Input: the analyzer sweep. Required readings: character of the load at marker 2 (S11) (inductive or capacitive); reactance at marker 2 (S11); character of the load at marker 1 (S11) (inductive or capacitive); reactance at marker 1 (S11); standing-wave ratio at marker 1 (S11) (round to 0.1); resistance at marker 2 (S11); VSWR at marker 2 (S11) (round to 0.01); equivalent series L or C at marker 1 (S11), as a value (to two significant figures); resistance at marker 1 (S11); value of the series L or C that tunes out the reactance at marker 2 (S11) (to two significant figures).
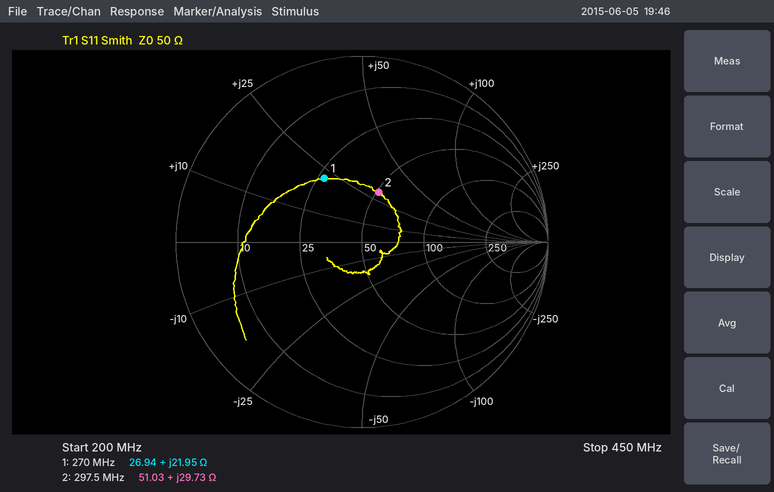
inductive
+29.73 Ω
inductive
+21.95 Ω
2.3
51.03 Ω
1.79
13 nH
26.94 Ω
18 pF
